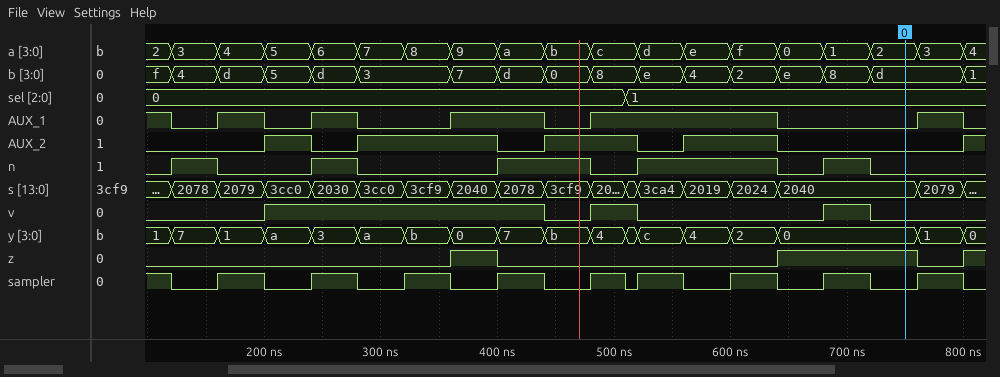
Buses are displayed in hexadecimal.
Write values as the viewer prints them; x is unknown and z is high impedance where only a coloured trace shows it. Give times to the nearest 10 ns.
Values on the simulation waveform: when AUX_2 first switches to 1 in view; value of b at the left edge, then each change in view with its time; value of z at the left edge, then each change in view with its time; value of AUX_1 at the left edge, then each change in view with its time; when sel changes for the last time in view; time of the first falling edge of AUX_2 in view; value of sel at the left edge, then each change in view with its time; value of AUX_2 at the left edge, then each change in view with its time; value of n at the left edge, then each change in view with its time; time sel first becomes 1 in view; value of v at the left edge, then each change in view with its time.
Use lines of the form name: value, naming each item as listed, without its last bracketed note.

when AUX_2 first switches to 1 in view: 200 ns
value of b at the left edge, then each change in view with its time: f, 4 at 120 ns, d at 160 ns, 5 at 200 ns, d at 240 ns, 3 at 280 ns, 7 at 360 ns, d at 400 ns, 0 at 440 ns, 8 at 480 ns, e at 520 ns, 4 at 560 ns, 2 at 600 ns, e at 640 ns, 8 at 680 ns, d at 720 ns, 1 at 800 ns
value of z at the left edge, then each change in view with its time: 0, 1 at 360 ns, 0 at 400 ns, 1 at 640 ns, 0 at 760 ns, 1 at 800 ns
value of AUX_1 at the left edge, then each change in view with its time: 1, 0 at 120 ns, 1 at 160 ns, 0 at 200 ns, 1 at 240 ns, 0 at 280 ns, 1 at 360 ns, 0 at 440 ns, 1 at 480 ns, 0 at 640 ns, 1 at 760 ns, 0 at 800 ns
when sel changes for the last time in view: 510 ns
time of the first falling edge of AUX_2 in view: 240 ns
value of sel at the left edge, then each change in view with its time: 0, 1 at 510 ns
value of AUX_2 at the left edge, then each change in view with its time: 0, 1 at 200 ns, 0 at 240 ns, 1 at 280 ns, 0 at 400 ns, 1 at 440 ns, 0 at 520 ns, 1 at 560 ns, 0 at 640 ns, 1 at 800 ns
value of n at the left edge, then each change in view with its time: 0, 1 at 120 ns, 0 at 160 ns, 1 at 240 ns, 0 at 280 ns, 1 at 400 ns, 0 at 480 ns, 1 at 520 ns, 0 at 640 ns, 1 at 680 ns, 0 at 720 ns
time sel first becomes 1 in view: 510 ns
value of v at the left edge, then each change in view with its time: 0, 1 at 200 ns, 0 at 440 ns, 1 at 480 ns, 0 at 520 ns, 1 at 680 ns, 0 at 720 ns
